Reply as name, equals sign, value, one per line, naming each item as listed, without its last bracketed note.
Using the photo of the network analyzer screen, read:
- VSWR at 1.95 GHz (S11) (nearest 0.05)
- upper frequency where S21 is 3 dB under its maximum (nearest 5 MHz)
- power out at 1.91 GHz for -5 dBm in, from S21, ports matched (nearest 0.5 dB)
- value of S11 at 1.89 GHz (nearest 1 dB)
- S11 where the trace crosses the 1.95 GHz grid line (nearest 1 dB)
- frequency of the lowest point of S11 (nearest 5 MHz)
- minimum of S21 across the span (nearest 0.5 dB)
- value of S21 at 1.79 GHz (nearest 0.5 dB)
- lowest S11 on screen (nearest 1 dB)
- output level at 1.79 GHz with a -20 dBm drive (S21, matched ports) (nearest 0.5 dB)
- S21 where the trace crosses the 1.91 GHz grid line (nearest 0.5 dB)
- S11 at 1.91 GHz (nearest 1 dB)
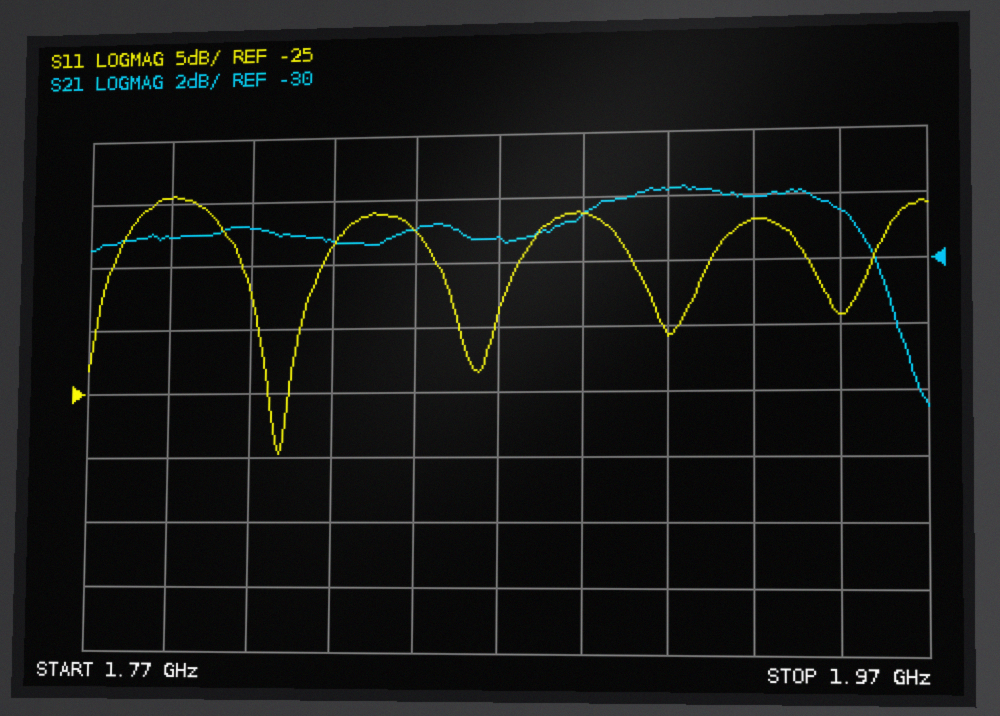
VSWR at 1.95 GHz (S11) = 1.25
upper frequency where S21 is 3 dB under its maximum = 1.960 GHz
power out at 1.91 GHz for -5 dBm in, from S21, ports matched = -33.0 dBm
value of S11 at 1.89 GHz = -11 dB
S11 where the trace crosses the 1.95 GHz grid line = -19 dB
frequency of the lowest point of S11 = 1.815 GHz
minimum of S21 across the span = -34.5 dB
value of S21 at 1.79 GHz = -29.0 dB
lowest S11 on screen = -30 dB
output level at 1.79 GHz with a -20 dBm drive (S21, matched ports) = -49.0 dBm
S21 where the trace crosses the 1.91 GHz grid line = -28.0 dB
S11 at 1.91 GHz = -21 dB
